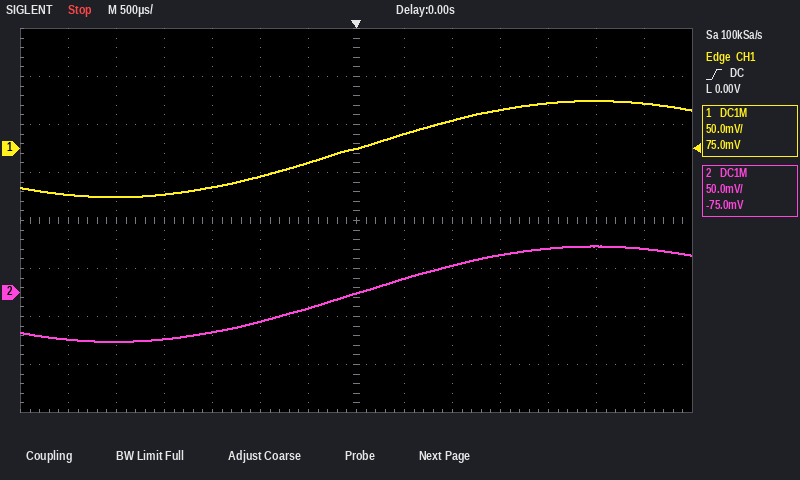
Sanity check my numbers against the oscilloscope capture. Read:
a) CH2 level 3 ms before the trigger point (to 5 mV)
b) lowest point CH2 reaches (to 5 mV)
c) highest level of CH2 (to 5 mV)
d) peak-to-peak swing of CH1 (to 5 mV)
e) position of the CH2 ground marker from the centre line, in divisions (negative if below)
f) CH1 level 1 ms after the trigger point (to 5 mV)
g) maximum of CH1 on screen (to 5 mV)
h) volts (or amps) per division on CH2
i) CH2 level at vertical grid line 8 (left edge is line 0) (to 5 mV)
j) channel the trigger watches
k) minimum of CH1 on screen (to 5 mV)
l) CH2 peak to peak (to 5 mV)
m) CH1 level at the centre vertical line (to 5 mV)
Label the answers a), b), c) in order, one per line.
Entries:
a) -50 mV
b) -50 mV
c) 50 mV
d) 100 mV
e) -1.5 div
f) 30 mV
g) 50 mV
h) 50 mV
i) 15 mV
j) CH1
k) -50 mV
l) 100 mV
m) 0 mV
